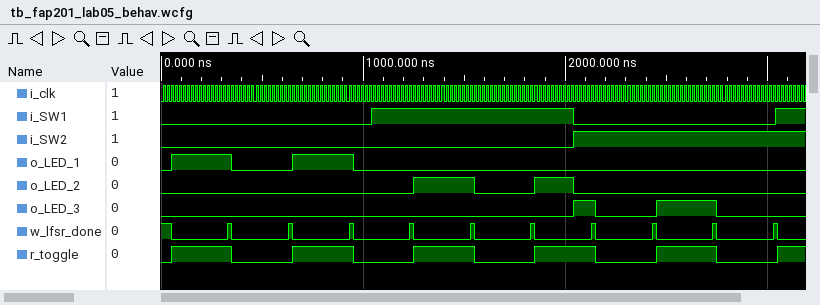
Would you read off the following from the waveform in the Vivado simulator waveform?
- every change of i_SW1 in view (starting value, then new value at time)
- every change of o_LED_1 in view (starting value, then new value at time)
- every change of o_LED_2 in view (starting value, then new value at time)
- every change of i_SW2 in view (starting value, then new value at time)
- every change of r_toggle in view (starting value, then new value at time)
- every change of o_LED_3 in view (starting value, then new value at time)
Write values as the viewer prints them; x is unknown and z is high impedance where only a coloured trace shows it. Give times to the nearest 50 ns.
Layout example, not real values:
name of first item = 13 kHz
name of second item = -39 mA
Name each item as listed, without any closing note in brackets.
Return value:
every change of i_SW1 in view = 0, 1 at 1050 ns, 0 at 2050 ns, 1 at 3050 ns
every change of o_LED_1 in view = 0, 1 at 50 ns, 0 at 350 ns, 1 at 650 ns, 0 at 950 ns
every change of o_LED_2 in view = 0, 1 at 1250 ns, 0 at 1550 ns, 1 at 1850 ns, 0 at 2050 ns
every change of i_SW2 in view = 0, 1 at 2050 ns
every change of r_toggle in view = 0, 1 at 50 ns, 0 at 350 ns, 1 at 650 ns, 0 at 950 ns, 1 at 1250 ns, 0 at 1550 ns, 1 at 1850 ns, 0 at 2150 ns, 1 at 2450 ns, 0 at 2750 ns, 1 at 3050 ns
every change of o_LED_3 in view = 0, 1 at 2050 ns, 0 at 2150 ns, 1 at 2450 ns, 0 at 2750 ns
